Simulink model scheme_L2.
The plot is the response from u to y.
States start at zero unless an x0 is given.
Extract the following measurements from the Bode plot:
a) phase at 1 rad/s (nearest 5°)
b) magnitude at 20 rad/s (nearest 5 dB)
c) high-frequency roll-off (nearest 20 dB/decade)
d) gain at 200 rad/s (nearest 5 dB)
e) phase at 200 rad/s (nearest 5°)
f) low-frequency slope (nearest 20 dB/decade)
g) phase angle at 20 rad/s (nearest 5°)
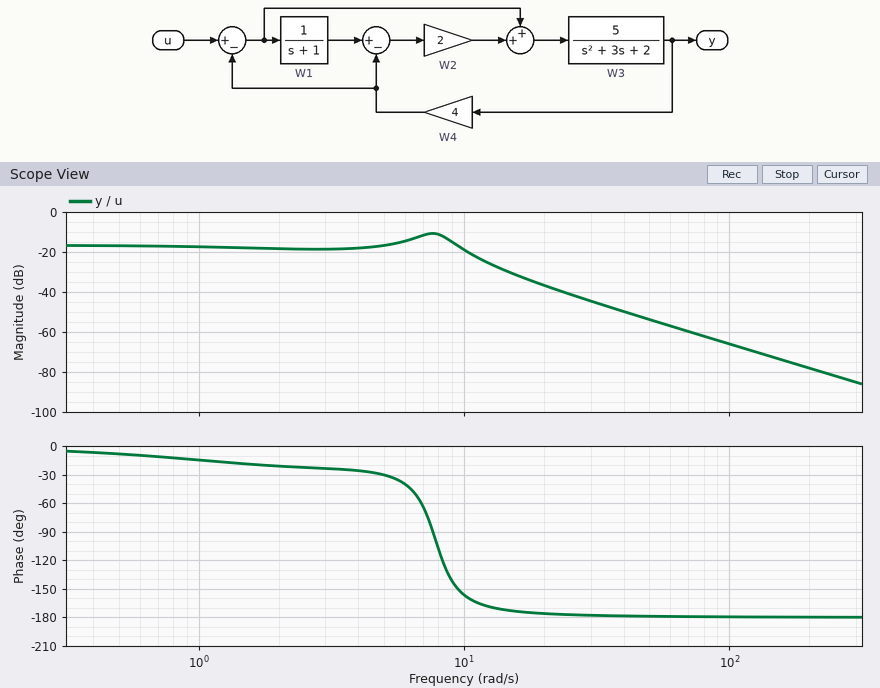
-15°
-35 dB
-40 dB/decade
-80 dB
-180°
0 dB/decade
-175°
